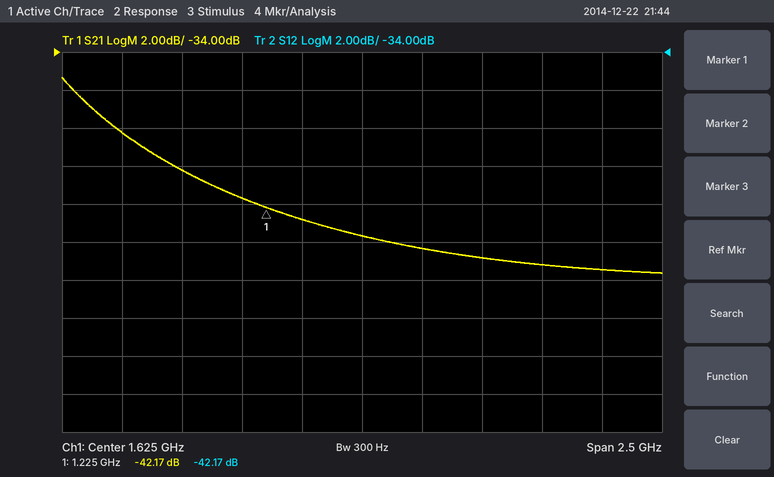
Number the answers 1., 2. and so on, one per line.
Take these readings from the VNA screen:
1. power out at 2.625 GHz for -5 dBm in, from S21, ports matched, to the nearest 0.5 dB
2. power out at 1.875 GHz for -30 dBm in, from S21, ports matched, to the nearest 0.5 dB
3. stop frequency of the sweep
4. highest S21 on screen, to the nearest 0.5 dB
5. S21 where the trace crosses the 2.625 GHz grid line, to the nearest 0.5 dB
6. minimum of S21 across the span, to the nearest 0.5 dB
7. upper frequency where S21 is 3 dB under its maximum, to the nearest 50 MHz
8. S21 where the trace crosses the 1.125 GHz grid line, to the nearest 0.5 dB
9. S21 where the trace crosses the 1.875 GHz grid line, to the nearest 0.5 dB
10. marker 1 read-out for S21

1. -50.5 dBm
2. -74.5 dBm
3. 2.875 GHz
4. -35.5 dB
5. -45.5 dB
6. -45.5 dB
7. 650 MHz
8. -41.5 dB
9. -44.5 dB
10. -42.17 dB
